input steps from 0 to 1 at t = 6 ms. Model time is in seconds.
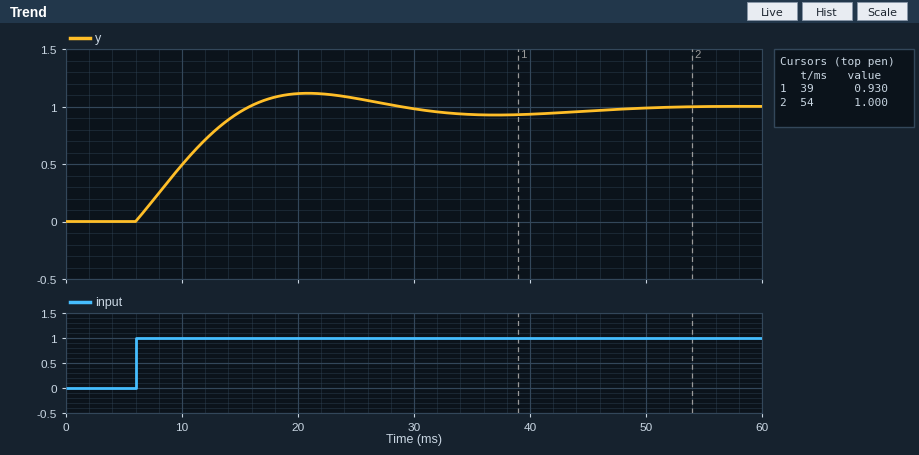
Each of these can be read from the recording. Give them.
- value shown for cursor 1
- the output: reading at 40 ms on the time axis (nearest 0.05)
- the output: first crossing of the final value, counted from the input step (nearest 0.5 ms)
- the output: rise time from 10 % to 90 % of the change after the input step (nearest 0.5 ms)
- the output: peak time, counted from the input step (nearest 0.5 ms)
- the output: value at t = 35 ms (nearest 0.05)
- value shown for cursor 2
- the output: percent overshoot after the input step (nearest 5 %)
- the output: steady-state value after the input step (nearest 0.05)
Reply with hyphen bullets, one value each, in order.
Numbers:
- 0.930
- 0.95
- 10.0 ms
- 7.5 ms
- 15.0 ms
- 0.95
- 1.000
- 10 %
- 1.00
